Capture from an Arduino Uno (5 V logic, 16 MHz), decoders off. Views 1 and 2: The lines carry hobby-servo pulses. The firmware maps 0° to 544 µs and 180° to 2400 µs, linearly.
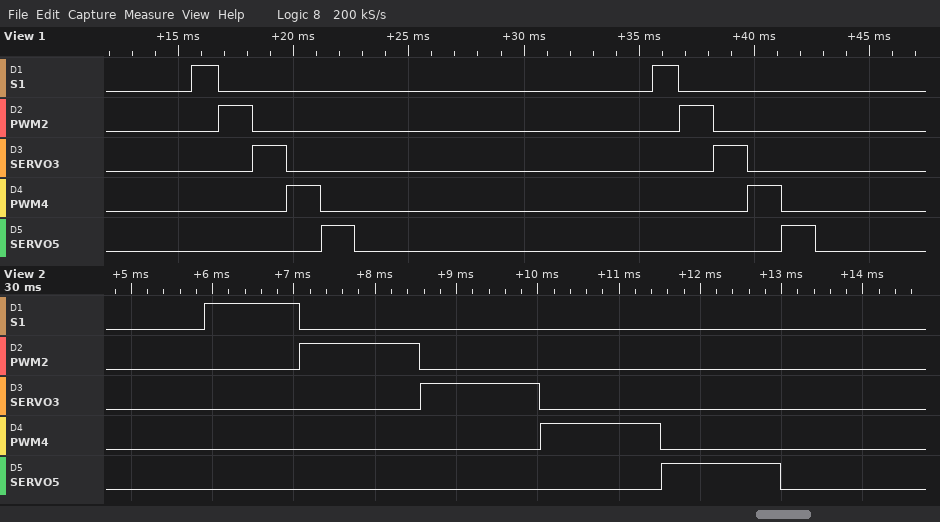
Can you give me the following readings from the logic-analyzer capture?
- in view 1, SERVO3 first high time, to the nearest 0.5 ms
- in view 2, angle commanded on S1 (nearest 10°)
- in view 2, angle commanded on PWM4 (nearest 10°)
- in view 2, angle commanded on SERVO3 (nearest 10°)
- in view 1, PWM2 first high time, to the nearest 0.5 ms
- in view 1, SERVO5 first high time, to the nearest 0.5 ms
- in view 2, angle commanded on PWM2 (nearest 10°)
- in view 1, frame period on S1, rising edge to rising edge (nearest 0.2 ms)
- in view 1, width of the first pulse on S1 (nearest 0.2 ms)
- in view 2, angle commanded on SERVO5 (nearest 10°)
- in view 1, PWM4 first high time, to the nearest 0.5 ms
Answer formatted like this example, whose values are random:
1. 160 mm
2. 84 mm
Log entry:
1. 1.5 ms
2. 60°
3. 90°
4. 90°
5. 1.5 ms
6. 1.5 ms
7. 90°
8. 20.0 ms
9. 1.2 ms
10. 90°
11. 1.5 ms
